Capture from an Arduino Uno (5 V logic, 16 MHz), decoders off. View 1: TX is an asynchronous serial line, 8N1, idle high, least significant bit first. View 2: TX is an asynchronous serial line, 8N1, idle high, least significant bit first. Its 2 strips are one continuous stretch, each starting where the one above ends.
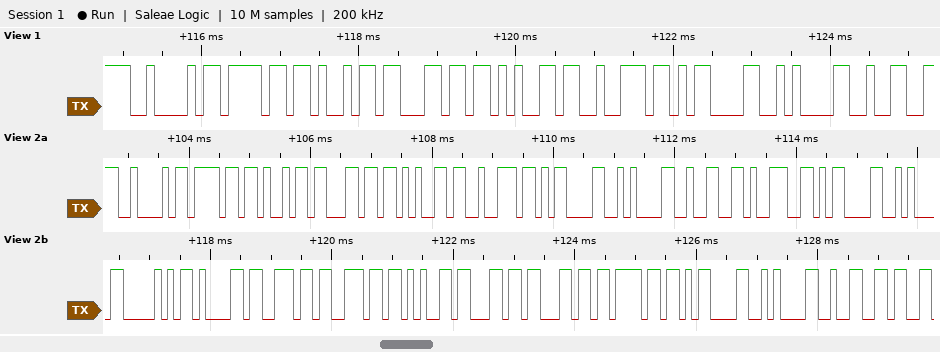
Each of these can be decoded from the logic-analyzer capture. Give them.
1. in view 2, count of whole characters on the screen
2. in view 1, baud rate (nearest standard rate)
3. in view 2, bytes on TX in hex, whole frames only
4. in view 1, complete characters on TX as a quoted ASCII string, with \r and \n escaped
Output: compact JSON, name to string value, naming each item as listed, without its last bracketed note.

{"in view 2, count of whole characters on the screen": "23", "in view 1, baud rate": "9600 baud", "in view 2, bytes on TX in hex, whole frames only": "42 6F 69 6C 65 72 0D 0A 32 39 0D 0A 50 61 6E 6E 65 6C 6C 6F 0D 0A 32", "in view 1, complete characters on TX as a quoted ASCII string, with \\r and \\n escaped": "\"Boiler\\r\\n2\""}
